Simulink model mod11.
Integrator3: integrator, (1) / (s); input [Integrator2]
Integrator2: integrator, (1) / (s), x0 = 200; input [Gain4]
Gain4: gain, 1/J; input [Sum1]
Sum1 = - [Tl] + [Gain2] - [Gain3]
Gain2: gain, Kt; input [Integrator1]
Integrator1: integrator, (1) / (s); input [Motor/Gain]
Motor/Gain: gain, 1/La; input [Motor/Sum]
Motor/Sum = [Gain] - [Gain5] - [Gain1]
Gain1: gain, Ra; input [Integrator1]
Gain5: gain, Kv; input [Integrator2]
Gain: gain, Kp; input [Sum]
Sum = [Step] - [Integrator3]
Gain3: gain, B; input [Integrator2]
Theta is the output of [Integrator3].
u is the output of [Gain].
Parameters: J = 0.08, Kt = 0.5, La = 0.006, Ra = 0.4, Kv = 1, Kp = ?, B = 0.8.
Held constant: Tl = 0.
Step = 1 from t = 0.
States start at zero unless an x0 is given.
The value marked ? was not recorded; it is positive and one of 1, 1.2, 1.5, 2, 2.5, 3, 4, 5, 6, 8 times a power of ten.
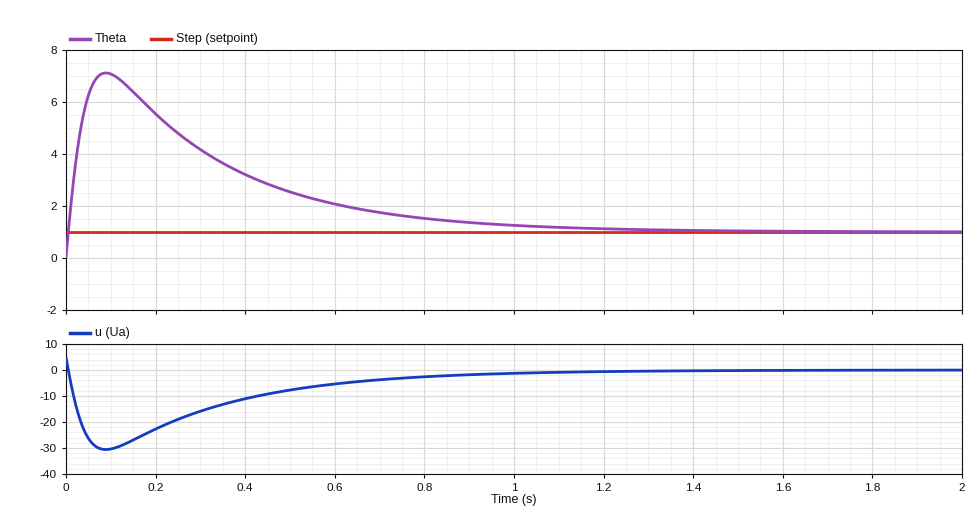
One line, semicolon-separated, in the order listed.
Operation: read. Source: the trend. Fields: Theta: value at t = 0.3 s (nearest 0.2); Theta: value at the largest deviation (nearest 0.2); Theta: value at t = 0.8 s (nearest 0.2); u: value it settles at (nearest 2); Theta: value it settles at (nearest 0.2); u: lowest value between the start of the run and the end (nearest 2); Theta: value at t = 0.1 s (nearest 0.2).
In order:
4.2; 7.2; 1.6; 0; 1.0; -30; 7.0
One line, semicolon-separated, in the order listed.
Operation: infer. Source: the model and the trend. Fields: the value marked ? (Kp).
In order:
5
